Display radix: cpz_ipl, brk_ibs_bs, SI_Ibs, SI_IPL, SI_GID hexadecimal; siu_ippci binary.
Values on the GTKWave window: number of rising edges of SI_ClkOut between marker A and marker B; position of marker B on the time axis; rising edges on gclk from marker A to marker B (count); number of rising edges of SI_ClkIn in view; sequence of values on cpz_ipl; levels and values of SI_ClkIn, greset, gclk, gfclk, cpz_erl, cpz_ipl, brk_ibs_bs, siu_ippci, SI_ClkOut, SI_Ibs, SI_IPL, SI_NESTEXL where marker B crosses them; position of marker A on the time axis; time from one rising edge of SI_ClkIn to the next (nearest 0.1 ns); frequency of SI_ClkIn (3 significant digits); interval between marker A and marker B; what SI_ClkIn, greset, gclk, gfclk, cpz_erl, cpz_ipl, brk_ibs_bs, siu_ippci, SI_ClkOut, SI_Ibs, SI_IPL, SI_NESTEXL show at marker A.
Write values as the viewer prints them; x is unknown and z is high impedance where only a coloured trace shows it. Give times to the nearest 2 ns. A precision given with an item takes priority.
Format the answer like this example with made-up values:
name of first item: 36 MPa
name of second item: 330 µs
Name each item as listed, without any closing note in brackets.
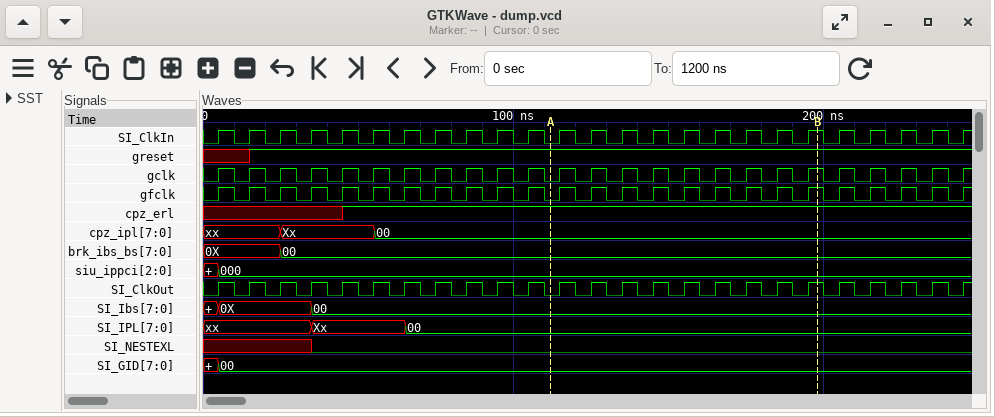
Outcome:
number of rising edges of SI_ClkOut between marker A and marker B: 9
position of marker B on the time axis: 198 ns
rising edges on gclk from marker A to marker B: 9
number of rising edges of SI_ClkIn in view: 25
sequence of values on cpz_ipl: xx, Xx, 00
levels and values of SI_ClkIn, greset, gclk, gfclk, cpz_erl, cpz_ipl, brk_ibs_bs, siu_ippci, SI_ClkOut, SI_Ibs, SI_IPL, SI_NESTEXL where marker B crosses them: SI_ClkIn=1, greset=1, gclk=1, gfclk=1, cpz_erl=1, cpz_ipl=00, brk_ibs_bs=00, siu_ippci=000, SI_ClkOut=1, SI_Ibs=00, SI_IPL=00, SI_NESTEXL=0
position of marker A on the time axis: 112 ns
time from one rising edge of SI_ClkIn to the next: 10 ns
frequency of SI_ClkIn: 100 MHz
interval between marker A and marker B: 86 ns
what SI_ClkIn, greset, gclk, gfclk, cpz_erl, cpz_ipl, brk_ibs_bs, siu_ippci, SI_ClkOut, SI_Ibs, SI_IPL, SI_NESTEXL show at marker A: SI_ClkIn=0, greset=1, gclk=0, gfclk=0, cpz_erl=1, cpz_ipl=00, brk_ibs_bs=00, siu_ippci=000, SI_ClkOut=0, SI_Ibs=00, SI_IPL=00, SI_NESTEXL=0
